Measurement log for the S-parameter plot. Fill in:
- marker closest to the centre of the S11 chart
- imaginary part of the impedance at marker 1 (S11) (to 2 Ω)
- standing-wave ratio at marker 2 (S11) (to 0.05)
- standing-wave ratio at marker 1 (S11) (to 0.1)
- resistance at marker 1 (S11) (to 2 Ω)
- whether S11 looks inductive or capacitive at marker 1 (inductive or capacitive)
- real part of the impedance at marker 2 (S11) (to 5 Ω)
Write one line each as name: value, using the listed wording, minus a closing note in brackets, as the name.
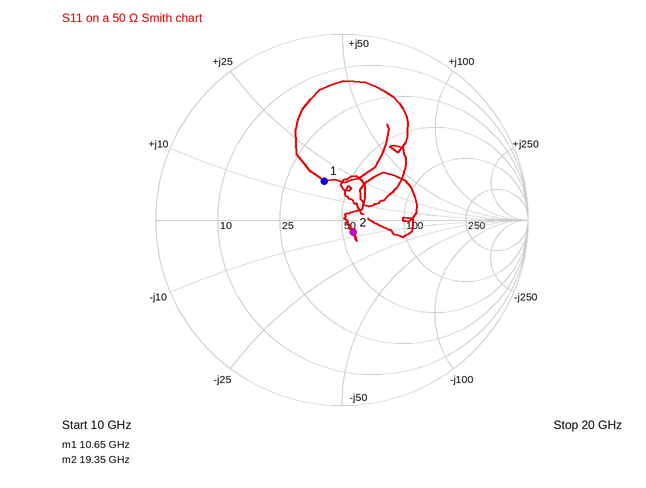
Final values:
marker closest to the centre of the S11 chart: marker 2
imaginary part of the impedance at marker 1 (S11): +16 Ω
standing-wave ratio at marker 2 (S11): 1.20
standing-wave ratio at marker 1 (S11): 1.6
resistance at marker 1 (S11): 38 Ω
whether S11 looks inductive or capacitive at marker 1: inductive
real part of the impedance at marker 2 (S11): 55 Ω
